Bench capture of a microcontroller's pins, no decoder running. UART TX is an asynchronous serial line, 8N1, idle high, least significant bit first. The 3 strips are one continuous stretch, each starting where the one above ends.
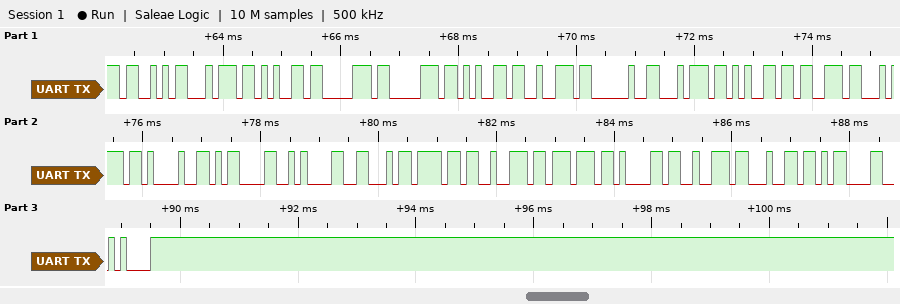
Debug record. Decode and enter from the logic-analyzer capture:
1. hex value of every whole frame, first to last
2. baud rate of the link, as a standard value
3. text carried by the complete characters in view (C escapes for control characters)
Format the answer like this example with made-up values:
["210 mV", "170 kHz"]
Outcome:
["0x53 0x74 0x65 0x70 0x70 0x65 0x72 0x20 0x74 0x65 0x73 0x74 0x21 0x0D 0x0A 0x46 0x6F 0x72 0x77 0x61 0x72 0x64 0x0D 0x0A", "9600 baud", "\"Stepper test!\\r\\nForward\\r\\n\""]
